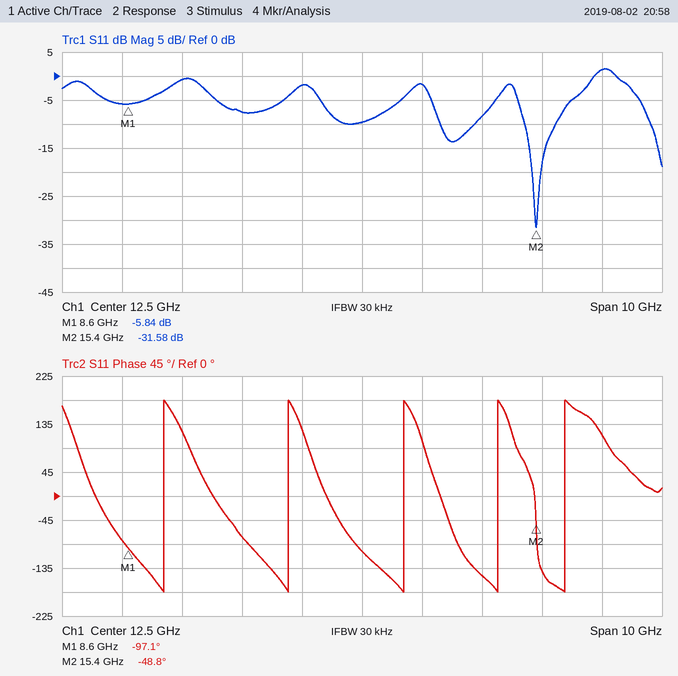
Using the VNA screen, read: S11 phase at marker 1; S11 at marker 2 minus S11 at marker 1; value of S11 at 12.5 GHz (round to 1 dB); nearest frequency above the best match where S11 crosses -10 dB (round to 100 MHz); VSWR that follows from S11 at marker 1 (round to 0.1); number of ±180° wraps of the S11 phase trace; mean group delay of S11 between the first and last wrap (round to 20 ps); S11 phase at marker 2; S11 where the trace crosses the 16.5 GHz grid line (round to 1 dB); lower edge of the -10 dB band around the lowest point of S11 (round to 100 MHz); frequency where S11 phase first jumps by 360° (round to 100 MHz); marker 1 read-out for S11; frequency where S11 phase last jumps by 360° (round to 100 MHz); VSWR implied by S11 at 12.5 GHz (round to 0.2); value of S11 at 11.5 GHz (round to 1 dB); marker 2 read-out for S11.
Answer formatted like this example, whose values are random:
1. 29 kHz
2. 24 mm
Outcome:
1. -97.1°
2. -25.74 dB
3. -10 dB
4. 15.7 GHz
5. 3.1
6. 5
7. 600 ps
8. -48.8°
9. 1 dB
10. 15.2 GHz
11. 9.2 GHz
12. -5.84 dB
13. 15.9 GHz
14. 2.0
15. -2 dB
16. -31.58 dB
